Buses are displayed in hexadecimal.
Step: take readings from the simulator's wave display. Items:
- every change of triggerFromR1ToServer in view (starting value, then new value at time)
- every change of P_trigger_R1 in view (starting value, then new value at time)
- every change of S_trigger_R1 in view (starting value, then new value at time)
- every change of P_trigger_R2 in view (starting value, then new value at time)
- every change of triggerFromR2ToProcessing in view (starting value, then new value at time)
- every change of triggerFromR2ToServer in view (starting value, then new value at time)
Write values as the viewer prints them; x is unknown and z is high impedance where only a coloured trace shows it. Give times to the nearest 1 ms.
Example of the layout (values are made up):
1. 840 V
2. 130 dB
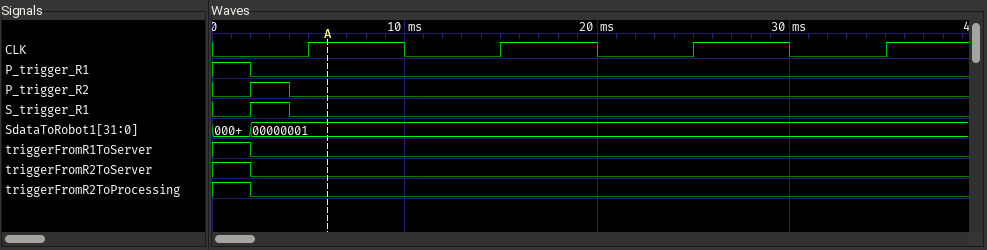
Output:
1. 1, 0 at 2 ms
2. 1, 0 at 2 ms
3. 0, 1 at 2 ms, 0 at 4 ms
4. 0, 1 at 2 ms, 0 at 4 ms
5. 1, 0 at 2 ms
6. 1, 0 at 2 ms
